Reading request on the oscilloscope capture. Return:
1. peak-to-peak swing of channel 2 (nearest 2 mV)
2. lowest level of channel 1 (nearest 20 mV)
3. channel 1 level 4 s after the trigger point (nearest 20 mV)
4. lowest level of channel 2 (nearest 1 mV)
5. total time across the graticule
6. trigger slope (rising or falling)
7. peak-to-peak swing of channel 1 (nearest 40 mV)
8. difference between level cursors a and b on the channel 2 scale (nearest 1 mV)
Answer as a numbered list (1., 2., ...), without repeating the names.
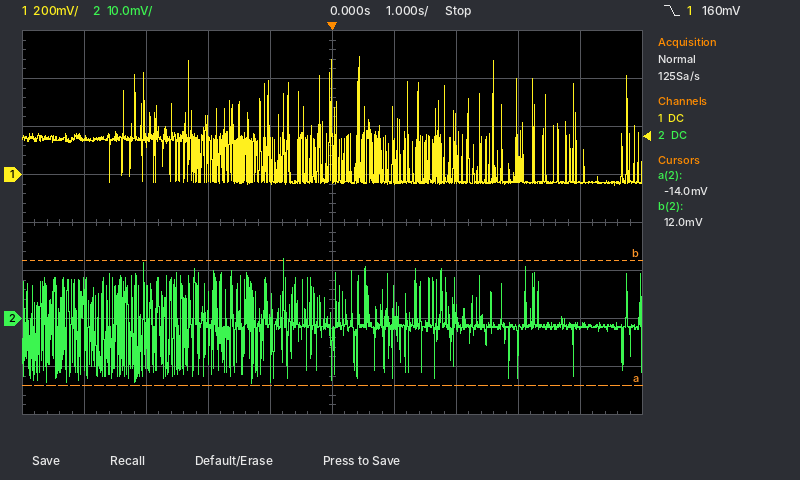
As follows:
1. 26 mV
2. -40 mV
3. -40 mV
4. -14 mV
5. 10 s
6. falling
7. 520 mV
8. 26 mV
